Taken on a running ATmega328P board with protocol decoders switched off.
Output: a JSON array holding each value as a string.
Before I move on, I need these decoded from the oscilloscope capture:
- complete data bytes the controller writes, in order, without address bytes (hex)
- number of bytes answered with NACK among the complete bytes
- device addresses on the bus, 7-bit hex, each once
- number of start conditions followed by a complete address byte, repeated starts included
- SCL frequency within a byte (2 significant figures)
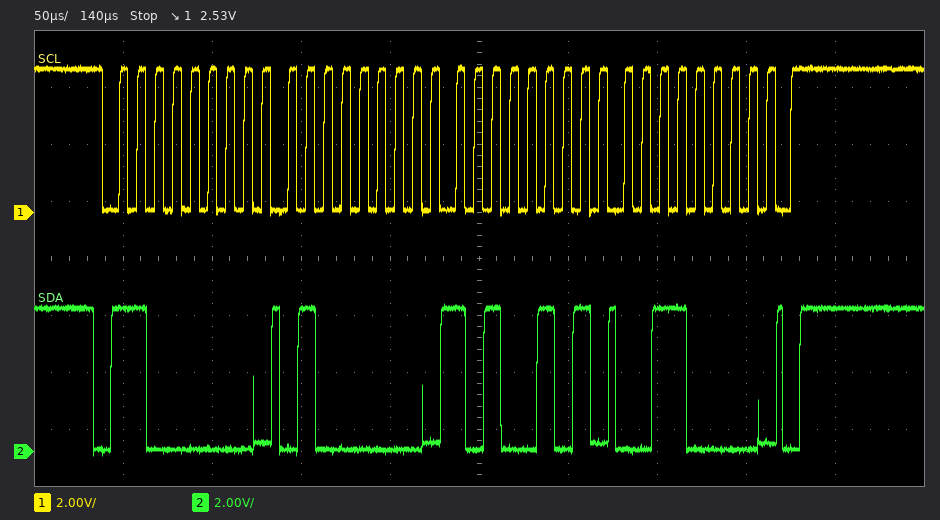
["40 A5 30", "0", "0x60", "1", "100 kHz"]
